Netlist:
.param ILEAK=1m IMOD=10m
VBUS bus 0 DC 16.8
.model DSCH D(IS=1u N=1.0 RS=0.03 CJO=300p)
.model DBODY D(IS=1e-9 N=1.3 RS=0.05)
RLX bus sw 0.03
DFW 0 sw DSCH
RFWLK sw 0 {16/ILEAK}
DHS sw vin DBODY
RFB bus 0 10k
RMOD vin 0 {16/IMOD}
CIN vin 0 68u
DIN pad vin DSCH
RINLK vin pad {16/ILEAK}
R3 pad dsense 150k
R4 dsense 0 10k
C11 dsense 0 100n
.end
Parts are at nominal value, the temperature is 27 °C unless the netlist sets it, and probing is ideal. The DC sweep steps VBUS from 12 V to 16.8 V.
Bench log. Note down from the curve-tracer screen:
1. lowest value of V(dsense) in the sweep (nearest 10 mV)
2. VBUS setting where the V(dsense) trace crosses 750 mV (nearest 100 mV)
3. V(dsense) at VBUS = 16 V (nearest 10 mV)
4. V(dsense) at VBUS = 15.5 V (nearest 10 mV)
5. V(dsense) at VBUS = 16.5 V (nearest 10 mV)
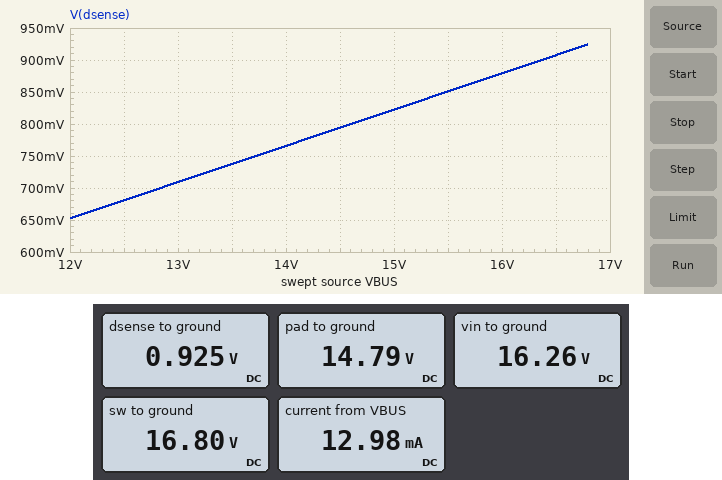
650 mV
13.7 V
880 mV
850 mV
910 mV
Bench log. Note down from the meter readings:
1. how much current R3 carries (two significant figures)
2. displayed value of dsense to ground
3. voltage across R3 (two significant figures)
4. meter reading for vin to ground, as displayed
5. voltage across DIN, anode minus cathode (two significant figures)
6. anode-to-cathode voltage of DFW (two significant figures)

92 µA
0.925 V
14 V
16.26 V
-1.5 V
-17 V
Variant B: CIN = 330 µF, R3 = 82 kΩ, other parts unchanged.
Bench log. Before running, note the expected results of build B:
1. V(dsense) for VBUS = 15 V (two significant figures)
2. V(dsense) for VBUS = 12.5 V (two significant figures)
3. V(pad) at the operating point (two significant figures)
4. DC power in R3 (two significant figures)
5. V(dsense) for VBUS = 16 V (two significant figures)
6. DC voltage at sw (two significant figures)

1.3 V
1.1 V
14 V
1.9 mW
1.4 V
17 V
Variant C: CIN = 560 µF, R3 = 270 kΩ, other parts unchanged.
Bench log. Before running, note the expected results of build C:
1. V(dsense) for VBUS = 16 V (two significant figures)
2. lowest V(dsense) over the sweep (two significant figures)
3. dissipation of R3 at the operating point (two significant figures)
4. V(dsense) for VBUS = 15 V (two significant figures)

520 mV
390 mV
820 µW
490 mV
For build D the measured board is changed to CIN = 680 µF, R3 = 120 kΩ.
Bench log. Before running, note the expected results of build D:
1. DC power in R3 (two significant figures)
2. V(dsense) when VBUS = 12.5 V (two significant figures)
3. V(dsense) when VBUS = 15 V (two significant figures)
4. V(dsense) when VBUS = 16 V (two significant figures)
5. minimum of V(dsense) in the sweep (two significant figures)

1.5 mW
820 mV
990 mV
1.1 V
790 mV
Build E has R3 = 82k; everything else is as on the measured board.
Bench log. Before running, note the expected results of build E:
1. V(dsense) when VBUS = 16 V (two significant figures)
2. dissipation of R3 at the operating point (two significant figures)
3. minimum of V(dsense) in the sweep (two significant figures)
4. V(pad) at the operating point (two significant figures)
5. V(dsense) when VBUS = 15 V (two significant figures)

1.4 V
1.9 mW
1.1 V
14 V
1.3 V
